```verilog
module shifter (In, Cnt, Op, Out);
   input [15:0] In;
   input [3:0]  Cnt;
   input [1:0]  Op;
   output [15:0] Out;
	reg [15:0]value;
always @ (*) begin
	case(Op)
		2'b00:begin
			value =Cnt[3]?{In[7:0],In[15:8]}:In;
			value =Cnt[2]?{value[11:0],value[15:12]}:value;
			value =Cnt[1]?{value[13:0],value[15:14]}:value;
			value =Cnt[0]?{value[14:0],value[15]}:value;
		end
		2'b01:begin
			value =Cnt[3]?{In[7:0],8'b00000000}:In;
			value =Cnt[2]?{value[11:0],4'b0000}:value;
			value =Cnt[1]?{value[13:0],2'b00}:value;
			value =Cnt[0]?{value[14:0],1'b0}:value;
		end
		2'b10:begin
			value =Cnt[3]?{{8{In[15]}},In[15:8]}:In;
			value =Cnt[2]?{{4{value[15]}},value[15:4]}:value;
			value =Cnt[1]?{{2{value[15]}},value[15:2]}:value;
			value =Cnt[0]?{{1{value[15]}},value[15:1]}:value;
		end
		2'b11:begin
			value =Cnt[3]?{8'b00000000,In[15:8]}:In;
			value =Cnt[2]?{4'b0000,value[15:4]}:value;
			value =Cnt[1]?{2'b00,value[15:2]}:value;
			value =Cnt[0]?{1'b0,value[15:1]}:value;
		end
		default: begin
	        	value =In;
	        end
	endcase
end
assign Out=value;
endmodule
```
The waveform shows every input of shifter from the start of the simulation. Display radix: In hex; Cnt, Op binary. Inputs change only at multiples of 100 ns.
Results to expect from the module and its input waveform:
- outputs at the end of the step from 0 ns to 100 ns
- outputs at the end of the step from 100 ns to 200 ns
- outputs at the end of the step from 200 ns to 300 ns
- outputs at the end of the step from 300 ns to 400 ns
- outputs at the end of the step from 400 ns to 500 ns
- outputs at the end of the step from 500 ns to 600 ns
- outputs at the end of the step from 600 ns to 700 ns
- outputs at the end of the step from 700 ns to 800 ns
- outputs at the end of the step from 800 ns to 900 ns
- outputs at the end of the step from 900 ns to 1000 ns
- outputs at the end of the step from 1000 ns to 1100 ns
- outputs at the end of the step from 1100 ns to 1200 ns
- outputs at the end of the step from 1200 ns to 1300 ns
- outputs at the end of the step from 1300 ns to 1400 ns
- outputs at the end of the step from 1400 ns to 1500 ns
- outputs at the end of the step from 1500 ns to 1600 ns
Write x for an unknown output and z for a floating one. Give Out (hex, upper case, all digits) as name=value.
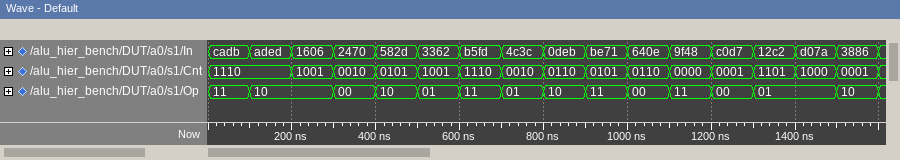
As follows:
Out=0003
Out=FFFE
Out=000B
Out=91C0
Out=02C1
Out=C400
Out=0002
Out=30F0
Out=0037
Out=05F3
Out=0399
Out=9F48
Out=81AF
Out=4000
Out=7A00
Out=1C43
